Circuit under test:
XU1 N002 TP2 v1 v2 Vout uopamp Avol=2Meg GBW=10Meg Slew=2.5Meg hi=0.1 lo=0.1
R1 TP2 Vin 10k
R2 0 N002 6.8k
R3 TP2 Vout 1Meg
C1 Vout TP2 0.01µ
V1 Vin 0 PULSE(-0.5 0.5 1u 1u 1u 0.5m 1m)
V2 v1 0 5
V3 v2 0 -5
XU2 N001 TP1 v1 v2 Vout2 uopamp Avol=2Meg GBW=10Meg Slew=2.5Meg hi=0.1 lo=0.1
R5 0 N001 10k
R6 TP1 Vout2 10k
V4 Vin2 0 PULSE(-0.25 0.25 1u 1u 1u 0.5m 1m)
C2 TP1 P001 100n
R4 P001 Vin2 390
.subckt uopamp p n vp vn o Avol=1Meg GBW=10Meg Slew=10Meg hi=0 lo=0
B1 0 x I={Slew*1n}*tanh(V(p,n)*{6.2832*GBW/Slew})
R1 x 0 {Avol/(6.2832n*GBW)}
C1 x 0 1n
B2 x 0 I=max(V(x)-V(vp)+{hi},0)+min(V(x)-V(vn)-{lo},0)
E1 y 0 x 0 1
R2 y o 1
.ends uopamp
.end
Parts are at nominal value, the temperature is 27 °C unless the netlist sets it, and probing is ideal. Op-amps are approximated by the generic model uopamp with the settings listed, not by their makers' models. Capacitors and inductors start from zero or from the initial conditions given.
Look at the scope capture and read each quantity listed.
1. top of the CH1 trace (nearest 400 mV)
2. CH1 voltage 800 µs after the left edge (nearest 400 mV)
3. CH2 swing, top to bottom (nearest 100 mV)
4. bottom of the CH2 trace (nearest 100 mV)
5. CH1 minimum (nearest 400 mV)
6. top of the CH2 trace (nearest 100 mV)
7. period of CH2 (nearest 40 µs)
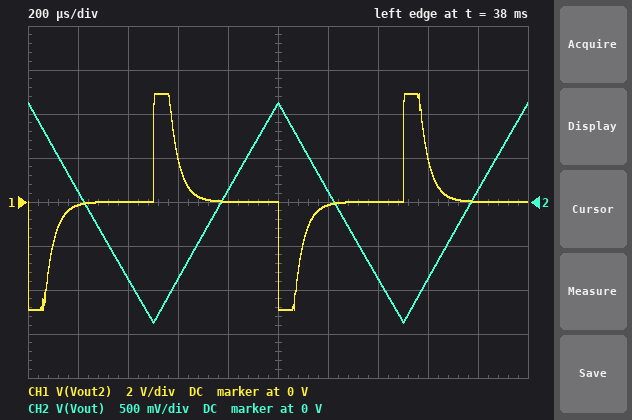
4.8 V
0 V
2.5 V
-1.4 V
-4.8 V
1.1 V
1.00 ms
